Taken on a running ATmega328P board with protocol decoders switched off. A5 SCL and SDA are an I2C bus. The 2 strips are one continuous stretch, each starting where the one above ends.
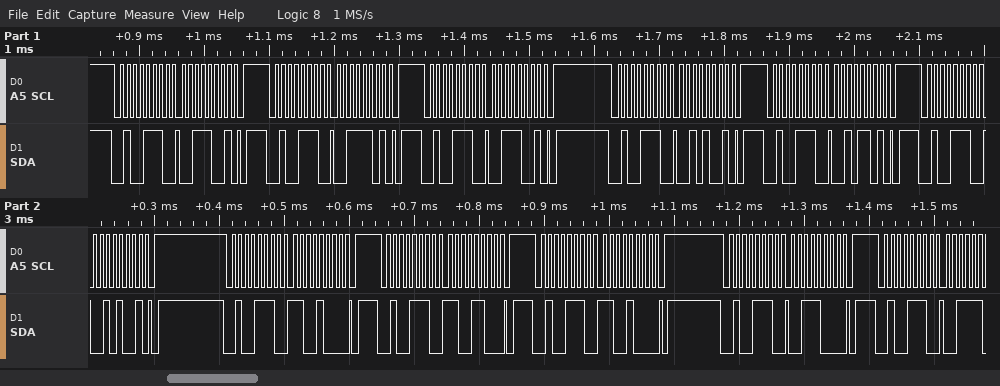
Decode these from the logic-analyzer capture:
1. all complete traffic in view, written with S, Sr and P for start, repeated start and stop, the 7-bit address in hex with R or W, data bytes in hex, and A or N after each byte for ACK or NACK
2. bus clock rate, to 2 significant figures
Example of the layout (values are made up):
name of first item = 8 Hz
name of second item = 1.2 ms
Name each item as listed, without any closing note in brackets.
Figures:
all complete traffic in view, written with S, Sr and P for start, repeated start and stop, the 7-bit address in hex with R or W, data bytes in hex, and A or N after each byte for ACK or NACK = S 27W A 39 A P S 27W A 3D A P S 27W A 39 A P S 27W A 29 A P S 27W A 2D A P S 27W A 29 A P S 27W A C8 A P S 27W A CC A P S 27W A C8 A P S 27W A 38 A P S 27W A
bus clock rate, to 2 significant figures = 100 kHz
